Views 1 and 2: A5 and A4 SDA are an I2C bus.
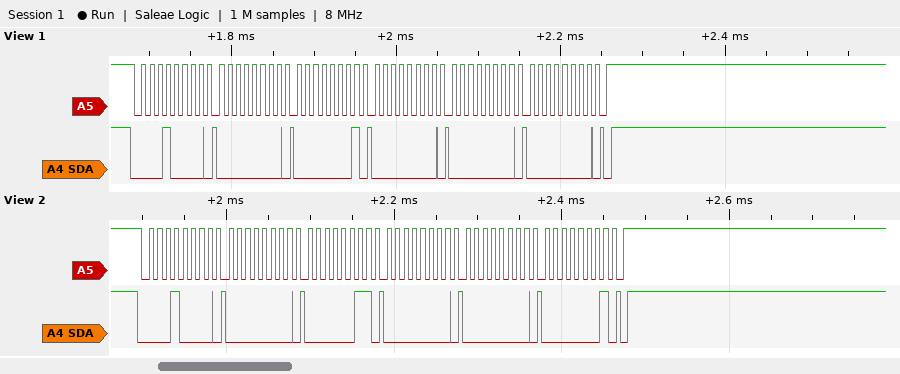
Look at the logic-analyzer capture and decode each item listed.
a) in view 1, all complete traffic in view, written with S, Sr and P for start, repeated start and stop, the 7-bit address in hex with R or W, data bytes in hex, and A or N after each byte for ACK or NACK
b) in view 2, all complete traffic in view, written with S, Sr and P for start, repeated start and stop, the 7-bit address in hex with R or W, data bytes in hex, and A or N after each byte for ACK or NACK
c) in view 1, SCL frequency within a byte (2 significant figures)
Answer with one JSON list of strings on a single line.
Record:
["S 08W A 00 A 01 A 00 A 00 A 00 A P", "S 08W A 00 A 03 A 00 A 00 A 01 A P", "100 kHz"]
